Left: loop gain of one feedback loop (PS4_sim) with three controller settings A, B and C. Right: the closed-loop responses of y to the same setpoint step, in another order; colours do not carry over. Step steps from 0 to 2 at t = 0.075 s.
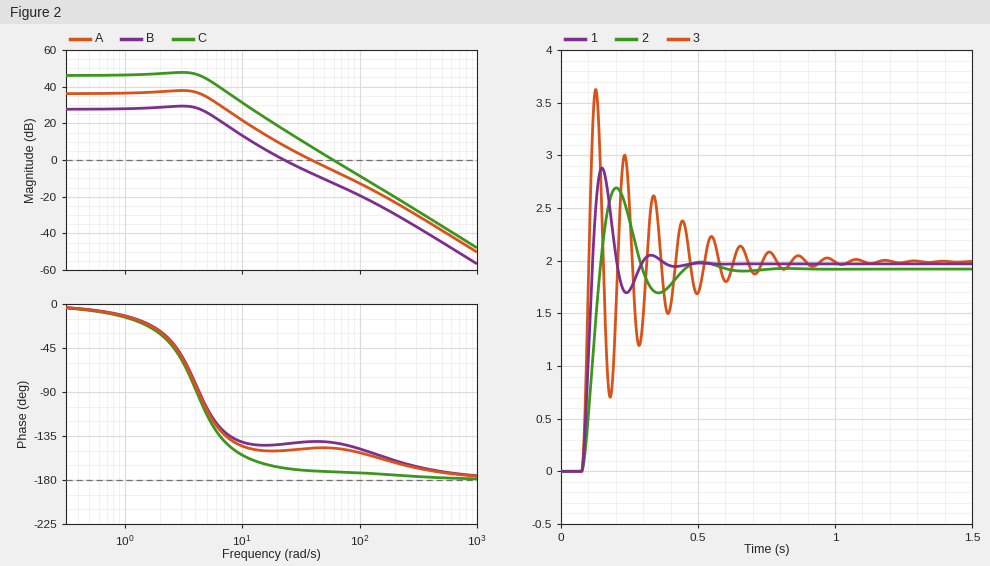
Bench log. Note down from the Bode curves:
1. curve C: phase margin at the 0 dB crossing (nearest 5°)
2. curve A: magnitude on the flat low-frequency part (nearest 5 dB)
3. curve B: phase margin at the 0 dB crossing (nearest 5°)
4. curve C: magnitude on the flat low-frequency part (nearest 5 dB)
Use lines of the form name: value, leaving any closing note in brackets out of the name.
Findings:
curve C: phase margin at the 0 dB crossing: 10°
curve A: magnitude on the flat low-frequency part: 35 dB
curve B: phase margin at the 0 dB crossing: 35°
curve C: magnitude on the flat low-frequency part: 45 dB
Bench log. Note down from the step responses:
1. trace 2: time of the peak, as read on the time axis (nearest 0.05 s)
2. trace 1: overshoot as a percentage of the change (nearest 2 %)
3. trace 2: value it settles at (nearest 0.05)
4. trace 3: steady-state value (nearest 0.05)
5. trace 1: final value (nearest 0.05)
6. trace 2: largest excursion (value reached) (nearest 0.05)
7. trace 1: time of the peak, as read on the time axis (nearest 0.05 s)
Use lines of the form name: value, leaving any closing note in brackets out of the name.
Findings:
trace 2: time of the peak, as read on the time axis: 0.20 s
trace 1: overshoot as a percentage of the change: 46 %
trace 2: value it settles at: 1.90
trace 3: steady-state value: 2.00
trace 1: final value: 1.95
trace 2: largest excursion (value reached): 2.70
trace 1: time of the peak, as read on the time axis: 0.15 s
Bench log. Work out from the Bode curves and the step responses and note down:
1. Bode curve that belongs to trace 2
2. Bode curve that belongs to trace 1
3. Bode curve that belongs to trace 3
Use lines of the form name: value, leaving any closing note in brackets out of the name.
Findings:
Bode curve that belongs to trace 2: B
Bode curve that belongs to trace 1: A
Bode curve that belongs to trace 3: C
